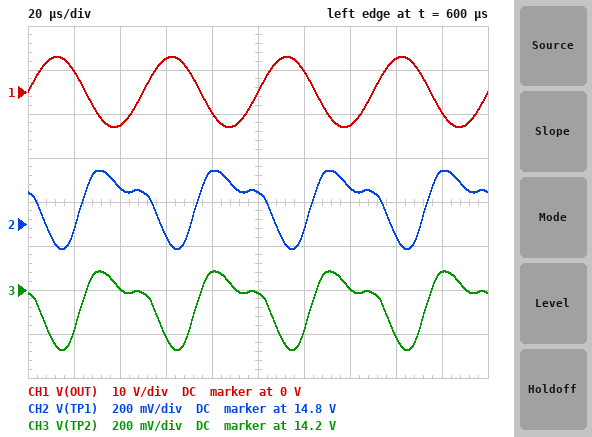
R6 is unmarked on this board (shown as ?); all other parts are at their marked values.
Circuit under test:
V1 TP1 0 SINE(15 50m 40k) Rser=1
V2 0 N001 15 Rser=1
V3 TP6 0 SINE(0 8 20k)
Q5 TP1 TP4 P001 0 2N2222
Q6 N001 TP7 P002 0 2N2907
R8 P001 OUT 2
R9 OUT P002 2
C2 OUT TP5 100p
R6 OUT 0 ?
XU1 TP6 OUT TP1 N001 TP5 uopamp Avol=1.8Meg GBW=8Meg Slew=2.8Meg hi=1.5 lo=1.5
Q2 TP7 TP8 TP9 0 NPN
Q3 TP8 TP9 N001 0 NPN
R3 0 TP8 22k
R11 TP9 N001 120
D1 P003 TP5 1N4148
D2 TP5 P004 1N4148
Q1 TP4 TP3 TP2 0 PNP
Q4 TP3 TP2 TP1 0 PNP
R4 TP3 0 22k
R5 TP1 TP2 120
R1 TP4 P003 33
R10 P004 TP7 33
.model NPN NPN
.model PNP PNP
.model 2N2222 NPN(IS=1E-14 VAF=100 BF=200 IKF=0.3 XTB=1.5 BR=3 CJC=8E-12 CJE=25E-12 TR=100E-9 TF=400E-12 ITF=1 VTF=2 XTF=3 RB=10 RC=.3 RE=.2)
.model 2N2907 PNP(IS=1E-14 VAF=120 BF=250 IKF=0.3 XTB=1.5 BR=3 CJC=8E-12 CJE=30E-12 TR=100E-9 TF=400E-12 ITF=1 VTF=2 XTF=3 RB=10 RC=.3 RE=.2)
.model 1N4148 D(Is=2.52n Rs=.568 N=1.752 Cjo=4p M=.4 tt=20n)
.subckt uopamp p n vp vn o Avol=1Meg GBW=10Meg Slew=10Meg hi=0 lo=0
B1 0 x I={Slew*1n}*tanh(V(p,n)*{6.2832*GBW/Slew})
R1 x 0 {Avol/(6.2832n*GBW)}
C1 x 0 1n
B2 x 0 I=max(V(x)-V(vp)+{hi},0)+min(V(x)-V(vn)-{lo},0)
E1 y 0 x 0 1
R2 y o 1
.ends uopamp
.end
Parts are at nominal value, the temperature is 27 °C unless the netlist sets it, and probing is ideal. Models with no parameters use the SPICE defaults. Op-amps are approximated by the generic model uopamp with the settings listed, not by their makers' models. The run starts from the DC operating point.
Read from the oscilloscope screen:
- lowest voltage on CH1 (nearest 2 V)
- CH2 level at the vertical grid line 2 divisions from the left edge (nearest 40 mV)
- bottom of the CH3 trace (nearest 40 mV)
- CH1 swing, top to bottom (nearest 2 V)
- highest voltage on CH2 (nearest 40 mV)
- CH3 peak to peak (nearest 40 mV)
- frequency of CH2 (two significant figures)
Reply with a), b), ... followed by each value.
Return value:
a) -8 V
b) 14.96 V
c) 13.92 V
d) 16 V
e) 15.04 V
f) 360 mV
g) 20 kHz
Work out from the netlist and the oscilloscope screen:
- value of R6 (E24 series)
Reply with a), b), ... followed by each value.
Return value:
a) 27 Ω
